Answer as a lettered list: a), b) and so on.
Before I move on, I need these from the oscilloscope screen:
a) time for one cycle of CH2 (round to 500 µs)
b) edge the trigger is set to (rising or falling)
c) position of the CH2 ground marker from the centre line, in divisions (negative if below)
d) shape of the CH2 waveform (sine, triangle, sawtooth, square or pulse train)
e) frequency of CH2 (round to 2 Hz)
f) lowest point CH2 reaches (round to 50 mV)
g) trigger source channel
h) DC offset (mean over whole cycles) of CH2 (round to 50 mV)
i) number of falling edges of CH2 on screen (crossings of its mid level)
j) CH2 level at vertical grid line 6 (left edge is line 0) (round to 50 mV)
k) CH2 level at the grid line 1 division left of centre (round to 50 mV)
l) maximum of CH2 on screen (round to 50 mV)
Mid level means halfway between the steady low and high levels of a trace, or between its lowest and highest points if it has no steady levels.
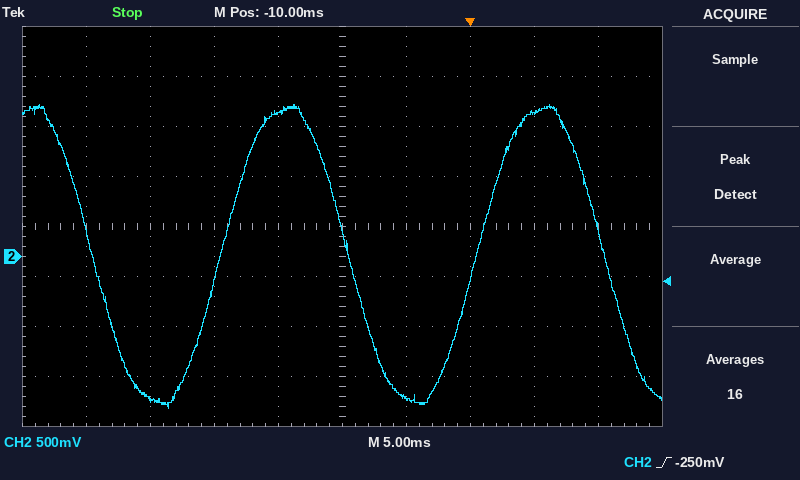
a) 20.0 ms
b) rising
c) -0.6 div
d) sine
e) 50 Hz
f) -1.50 V
g) CH2
h) 0 mV
i) 3
j) -1.40 V
k) 1.45 V
l) 1.50 V
